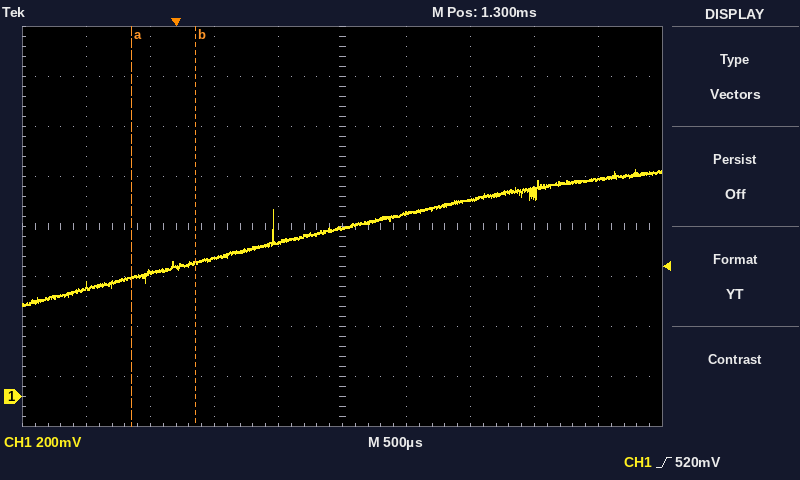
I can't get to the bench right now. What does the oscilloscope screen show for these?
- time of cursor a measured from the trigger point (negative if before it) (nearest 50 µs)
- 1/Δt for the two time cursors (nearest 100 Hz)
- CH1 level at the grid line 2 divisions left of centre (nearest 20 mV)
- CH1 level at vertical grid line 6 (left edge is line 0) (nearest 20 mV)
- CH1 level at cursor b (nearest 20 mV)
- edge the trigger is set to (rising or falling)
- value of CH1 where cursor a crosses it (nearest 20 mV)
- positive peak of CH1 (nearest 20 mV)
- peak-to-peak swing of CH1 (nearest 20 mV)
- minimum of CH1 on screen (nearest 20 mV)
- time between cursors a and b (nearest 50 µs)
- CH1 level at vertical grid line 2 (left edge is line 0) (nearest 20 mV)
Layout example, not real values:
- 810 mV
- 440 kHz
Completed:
- -350 µs
- 2.0 kHz
- 560 mV
- 740 mV
- 540 mV
- rising
- 480 mV
- 900 mV
- 540 mV
- 360 mV
- 500 µs
- 500 mV
